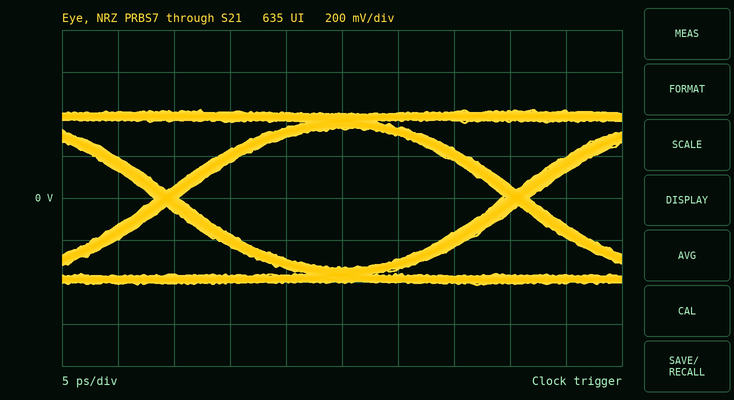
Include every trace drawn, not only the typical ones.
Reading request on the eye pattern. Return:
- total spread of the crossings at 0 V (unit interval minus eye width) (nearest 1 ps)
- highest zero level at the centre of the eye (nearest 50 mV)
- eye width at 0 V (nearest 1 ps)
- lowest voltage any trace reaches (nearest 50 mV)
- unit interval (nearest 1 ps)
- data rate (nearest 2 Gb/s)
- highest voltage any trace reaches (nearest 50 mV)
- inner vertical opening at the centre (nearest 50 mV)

2 ps
-350 mV
29 ps
-400 mV
31 ps
32 Gb/s
400 mV
650 mV
